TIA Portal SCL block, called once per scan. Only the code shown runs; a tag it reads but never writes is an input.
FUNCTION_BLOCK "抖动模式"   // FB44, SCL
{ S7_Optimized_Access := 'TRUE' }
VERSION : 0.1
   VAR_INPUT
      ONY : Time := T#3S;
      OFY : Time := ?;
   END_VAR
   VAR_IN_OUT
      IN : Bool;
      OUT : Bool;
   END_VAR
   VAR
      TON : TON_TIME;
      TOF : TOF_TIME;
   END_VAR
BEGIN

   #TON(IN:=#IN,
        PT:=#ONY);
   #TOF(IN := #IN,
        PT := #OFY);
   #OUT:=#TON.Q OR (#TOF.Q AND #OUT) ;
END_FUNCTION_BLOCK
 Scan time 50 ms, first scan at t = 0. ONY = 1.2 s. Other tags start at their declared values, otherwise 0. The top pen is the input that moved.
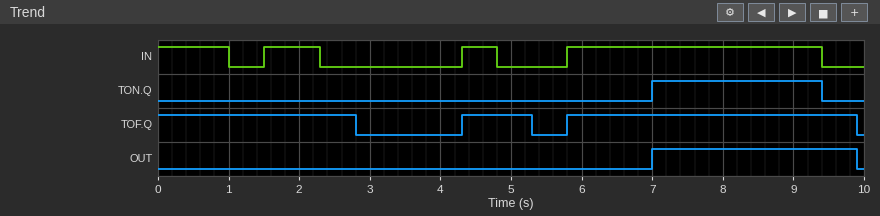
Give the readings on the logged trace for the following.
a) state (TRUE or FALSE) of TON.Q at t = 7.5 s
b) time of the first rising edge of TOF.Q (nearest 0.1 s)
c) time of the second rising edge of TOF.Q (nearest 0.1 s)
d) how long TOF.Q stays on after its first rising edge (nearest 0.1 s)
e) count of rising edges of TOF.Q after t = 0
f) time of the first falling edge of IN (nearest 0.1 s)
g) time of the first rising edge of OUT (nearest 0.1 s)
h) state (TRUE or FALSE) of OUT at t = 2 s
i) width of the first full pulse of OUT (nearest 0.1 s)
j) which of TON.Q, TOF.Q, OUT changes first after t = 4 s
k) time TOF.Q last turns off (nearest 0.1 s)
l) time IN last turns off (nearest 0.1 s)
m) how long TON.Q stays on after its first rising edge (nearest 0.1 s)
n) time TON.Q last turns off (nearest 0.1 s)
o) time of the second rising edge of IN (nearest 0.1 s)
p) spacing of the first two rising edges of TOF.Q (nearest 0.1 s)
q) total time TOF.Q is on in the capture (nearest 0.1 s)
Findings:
TRUE
4.3 s
5.8 s
1.0 s
2
1.0 s
7.0 s
FALSE
2.9 s
TOF.Q
9.9 s
9.4 s
2.4 s
9.4 s
4.3 s
1.5 s
7.9 s
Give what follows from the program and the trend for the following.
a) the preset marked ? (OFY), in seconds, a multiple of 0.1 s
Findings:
0.5 s
